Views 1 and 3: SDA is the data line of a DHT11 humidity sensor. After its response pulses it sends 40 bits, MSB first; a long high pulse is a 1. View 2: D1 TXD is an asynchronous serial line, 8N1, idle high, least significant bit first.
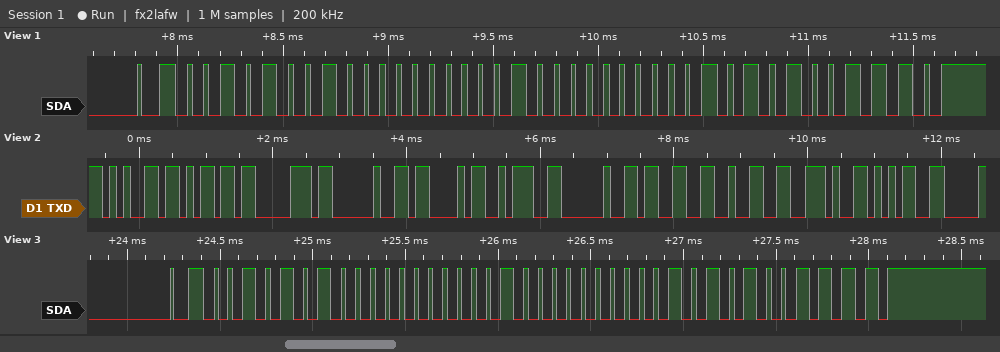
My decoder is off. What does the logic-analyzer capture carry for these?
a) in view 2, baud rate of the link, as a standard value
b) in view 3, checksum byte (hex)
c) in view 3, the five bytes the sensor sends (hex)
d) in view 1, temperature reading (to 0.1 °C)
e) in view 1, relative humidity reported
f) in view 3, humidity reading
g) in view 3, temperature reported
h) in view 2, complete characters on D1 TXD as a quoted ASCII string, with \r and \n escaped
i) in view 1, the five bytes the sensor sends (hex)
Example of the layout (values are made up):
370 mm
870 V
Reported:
9600 baud
0x4F
2A 00 20 05 4F
32.5 °C
41 %
42 %
32.5 °C
"emp C: 32.5"
29 00 20 05 4E
